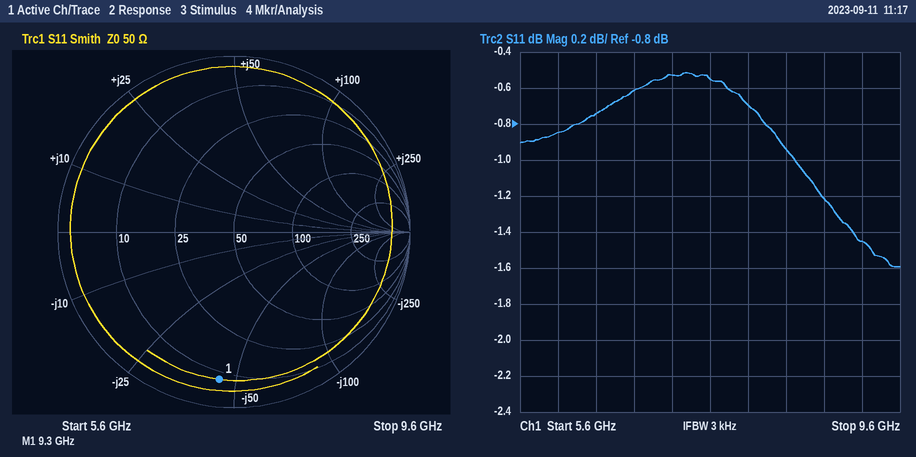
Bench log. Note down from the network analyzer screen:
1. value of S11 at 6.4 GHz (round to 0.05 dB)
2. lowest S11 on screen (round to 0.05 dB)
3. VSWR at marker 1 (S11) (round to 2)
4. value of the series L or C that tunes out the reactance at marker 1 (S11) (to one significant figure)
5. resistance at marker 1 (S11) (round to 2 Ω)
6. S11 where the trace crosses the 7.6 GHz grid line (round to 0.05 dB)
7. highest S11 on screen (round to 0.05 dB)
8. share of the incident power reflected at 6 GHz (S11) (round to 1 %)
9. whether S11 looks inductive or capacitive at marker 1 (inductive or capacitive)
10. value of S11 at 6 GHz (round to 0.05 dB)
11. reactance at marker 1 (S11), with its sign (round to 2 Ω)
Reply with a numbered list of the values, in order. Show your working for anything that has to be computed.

1. -0.75 dB
2. -1.60 dB
3. 12
4. L = 44 Ω/(2π × 9.3 GHz) ≈ 753 pH, so 800 pH to one significant figure
5. 8 Ω
6. -0.55 dB
7. -0.50 dB
8. 10^(-0.85/10) ≈ 82 %
9. capacitive
10. -0.85 dB
11. -44 Ω
